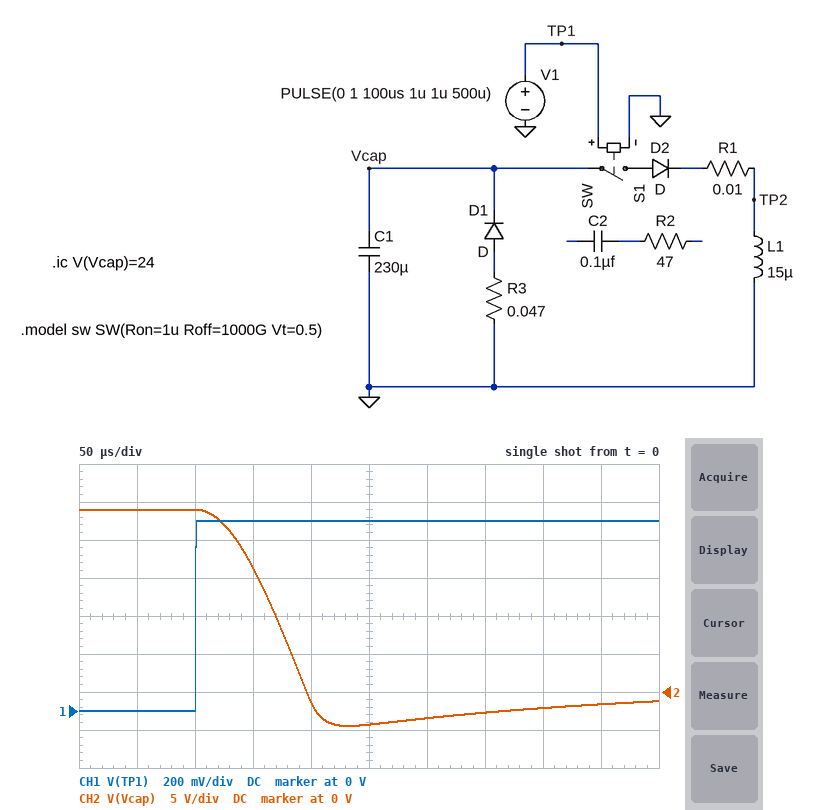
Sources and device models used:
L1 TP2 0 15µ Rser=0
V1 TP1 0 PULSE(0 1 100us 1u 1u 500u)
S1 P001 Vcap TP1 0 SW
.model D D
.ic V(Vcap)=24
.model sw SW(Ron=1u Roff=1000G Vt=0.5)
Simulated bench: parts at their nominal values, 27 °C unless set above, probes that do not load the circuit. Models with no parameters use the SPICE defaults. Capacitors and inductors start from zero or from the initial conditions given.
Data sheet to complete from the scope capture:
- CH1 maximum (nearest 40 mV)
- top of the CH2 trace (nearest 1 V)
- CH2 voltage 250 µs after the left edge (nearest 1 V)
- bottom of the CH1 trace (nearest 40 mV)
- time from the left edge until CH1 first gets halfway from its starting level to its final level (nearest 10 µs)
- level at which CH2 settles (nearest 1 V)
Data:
1.00 V
24 V
-4 V
0 V
100 µs
-1 V
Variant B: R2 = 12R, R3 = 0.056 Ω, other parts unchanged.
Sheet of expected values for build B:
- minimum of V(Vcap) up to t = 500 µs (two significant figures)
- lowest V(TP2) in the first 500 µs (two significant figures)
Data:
-5.0 V
-6.7 V
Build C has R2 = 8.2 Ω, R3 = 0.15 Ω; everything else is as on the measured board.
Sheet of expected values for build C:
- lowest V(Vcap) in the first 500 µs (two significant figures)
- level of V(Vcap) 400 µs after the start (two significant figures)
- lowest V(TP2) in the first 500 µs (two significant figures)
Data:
-9.2 V
-1.6 V
-11 V
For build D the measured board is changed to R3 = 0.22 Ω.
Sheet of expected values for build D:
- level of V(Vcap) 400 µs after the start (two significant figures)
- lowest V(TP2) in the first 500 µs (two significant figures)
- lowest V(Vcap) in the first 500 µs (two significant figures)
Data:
-2.2 V
-13 V
-11 V
